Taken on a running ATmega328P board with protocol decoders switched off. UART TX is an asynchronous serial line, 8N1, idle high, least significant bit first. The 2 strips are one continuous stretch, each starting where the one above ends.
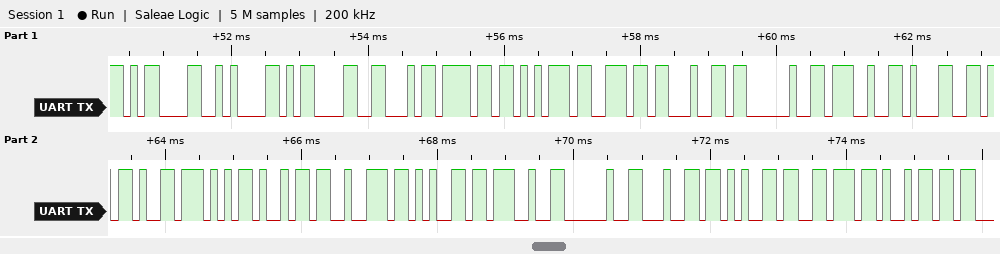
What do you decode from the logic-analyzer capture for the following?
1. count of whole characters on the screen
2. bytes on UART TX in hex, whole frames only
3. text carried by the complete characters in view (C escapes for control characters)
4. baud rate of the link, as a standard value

22
0D 0A 0D 46 6F 75 6E 64 20 27 31 2D 57 69 72 65 27 20 64 65 76 69
"\r\n\rFound '1-Wire' devi"
9600 baud
